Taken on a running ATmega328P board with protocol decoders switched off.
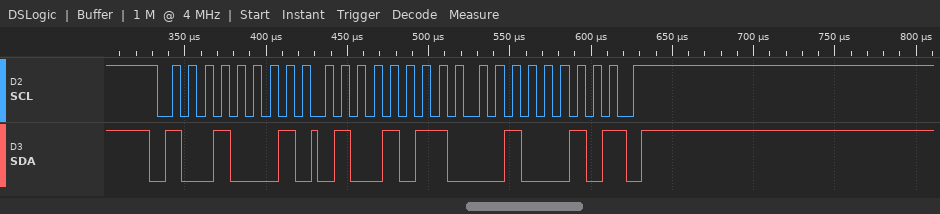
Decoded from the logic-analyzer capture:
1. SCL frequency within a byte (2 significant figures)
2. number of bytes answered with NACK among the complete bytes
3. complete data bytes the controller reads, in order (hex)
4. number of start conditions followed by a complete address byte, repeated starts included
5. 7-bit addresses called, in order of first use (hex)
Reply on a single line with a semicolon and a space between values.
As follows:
100 kHz; 1; 4B 22; 1; 0x48
